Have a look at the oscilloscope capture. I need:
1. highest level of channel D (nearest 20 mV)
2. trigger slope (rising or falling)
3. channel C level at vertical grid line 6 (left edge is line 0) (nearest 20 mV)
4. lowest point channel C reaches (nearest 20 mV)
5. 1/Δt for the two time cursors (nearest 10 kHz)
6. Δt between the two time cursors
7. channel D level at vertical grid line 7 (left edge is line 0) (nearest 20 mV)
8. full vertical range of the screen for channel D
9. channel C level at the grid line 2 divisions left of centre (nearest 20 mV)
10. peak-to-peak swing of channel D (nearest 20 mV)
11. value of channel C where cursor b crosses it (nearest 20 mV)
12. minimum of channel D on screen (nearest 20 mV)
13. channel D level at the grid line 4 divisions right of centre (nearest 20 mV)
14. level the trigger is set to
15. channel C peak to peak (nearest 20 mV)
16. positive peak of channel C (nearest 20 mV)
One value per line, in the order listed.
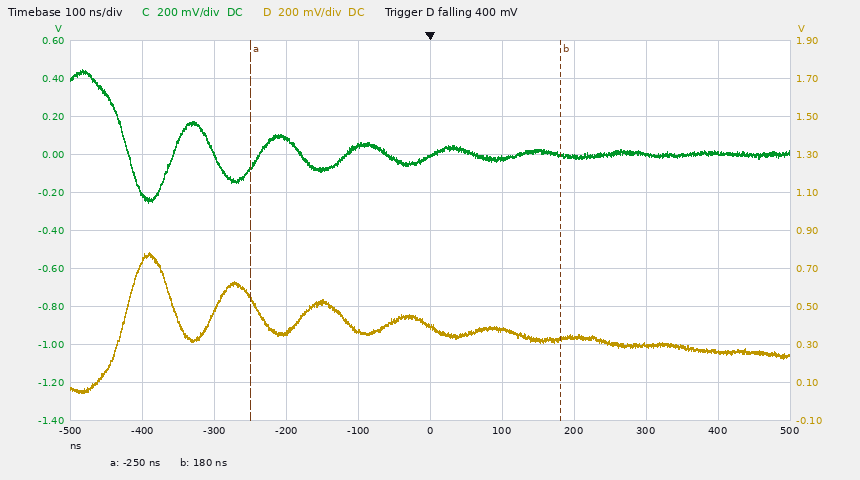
780 mV
falling
-20 mV
-260 mV
2.33 MHz
430 ns
340 mV
2 V
80 mV
740 mV
0 mV
40 mV
260 mV
400 mV
700 mV
440 mV
